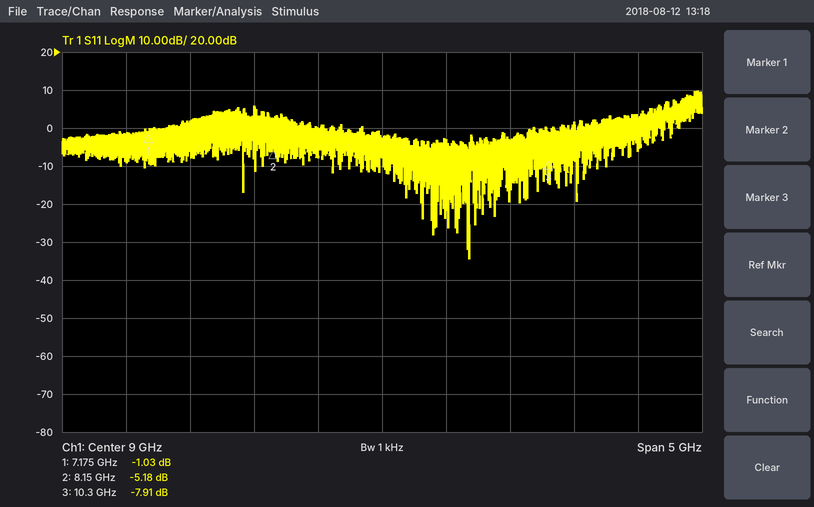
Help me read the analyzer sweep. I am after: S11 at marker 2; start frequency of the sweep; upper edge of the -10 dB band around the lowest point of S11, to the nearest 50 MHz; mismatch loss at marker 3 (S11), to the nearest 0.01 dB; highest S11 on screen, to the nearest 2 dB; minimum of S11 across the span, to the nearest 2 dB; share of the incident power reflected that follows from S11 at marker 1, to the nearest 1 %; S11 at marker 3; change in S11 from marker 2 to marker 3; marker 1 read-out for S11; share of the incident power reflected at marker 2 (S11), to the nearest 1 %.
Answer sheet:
-5.18 dB
6.5 GHz
9.70 GHz
0.77 dB
10 dB
-34 dB
79 %
-7.91 dB
-2.73 dB
-1.03 dB
30 %
